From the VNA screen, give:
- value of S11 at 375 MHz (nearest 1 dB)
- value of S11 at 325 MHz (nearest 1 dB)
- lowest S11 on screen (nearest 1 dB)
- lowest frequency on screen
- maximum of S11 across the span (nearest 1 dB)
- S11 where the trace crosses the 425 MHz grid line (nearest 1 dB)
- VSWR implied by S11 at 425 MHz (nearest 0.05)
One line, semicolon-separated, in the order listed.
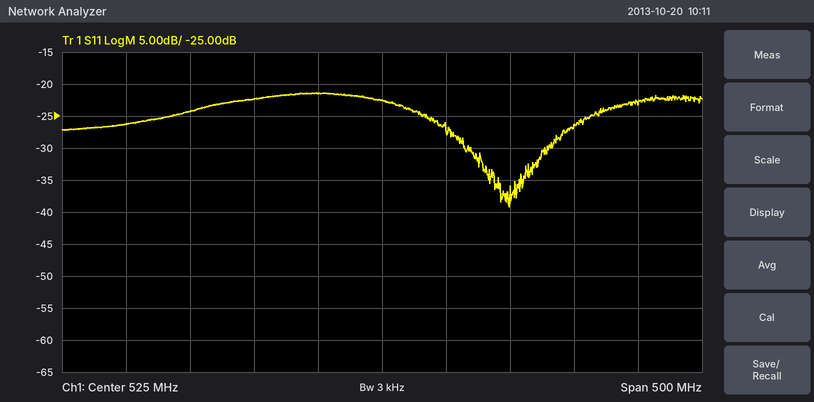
-24 dB; -26 dB; -39 dB; 275 MHz; -21 dB; -22 dB; 1.15
